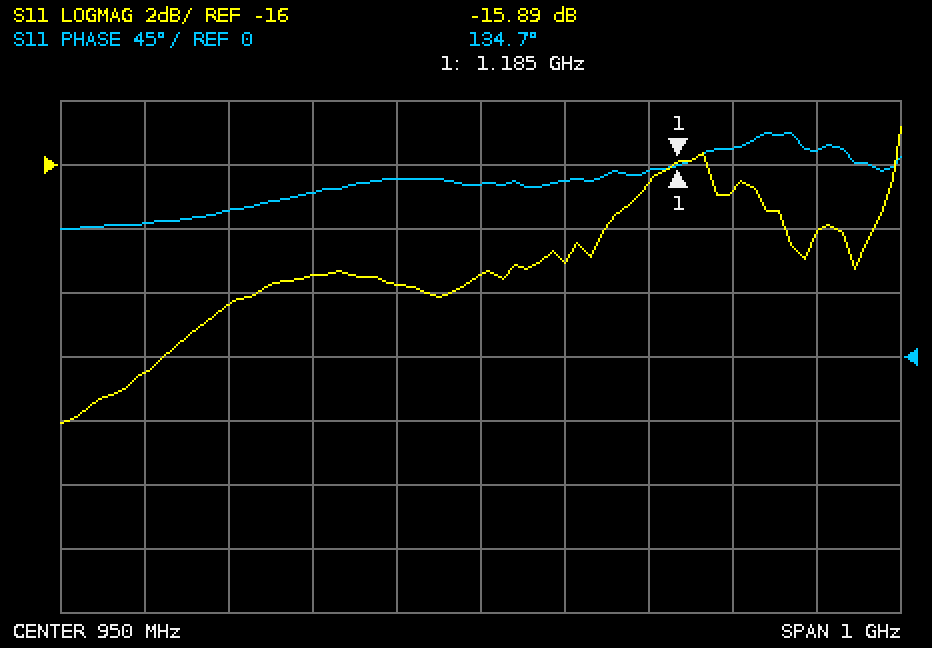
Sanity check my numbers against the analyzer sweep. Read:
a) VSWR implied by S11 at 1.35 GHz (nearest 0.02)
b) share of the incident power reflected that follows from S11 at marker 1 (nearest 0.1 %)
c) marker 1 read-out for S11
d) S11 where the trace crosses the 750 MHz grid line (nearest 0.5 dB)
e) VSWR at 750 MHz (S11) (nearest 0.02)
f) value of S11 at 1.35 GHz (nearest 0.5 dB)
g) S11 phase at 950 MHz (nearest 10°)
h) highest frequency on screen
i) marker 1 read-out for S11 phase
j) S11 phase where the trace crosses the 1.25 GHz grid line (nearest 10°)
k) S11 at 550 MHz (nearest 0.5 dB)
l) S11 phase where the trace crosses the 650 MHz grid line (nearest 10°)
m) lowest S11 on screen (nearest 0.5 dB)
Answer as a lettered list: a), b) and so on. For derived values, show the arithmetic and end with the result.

a) |Γ| = 10^(-18/20) = 0.1259; VSWR = (1 + 0.1259)/(1 − 0.1259) ≈ 1.29, so 1.28 to the nearest 0.02
b) 10^(-15.89/10) ≈ 2.6 %
c) -15.89 dB
d) -19.5 dB
e) |Γ| = 10^(-19.5/20) = 0.1059; VSWR = (1 + 0.1059)/(1 − 0.1059) ≈ 1.24
f) -18.0 dB
g) 120°
h) 1.45 GHz
i) 134.7°
j) 150°
k) -22.5 dB
l) 100°
m) -24.0 dB
